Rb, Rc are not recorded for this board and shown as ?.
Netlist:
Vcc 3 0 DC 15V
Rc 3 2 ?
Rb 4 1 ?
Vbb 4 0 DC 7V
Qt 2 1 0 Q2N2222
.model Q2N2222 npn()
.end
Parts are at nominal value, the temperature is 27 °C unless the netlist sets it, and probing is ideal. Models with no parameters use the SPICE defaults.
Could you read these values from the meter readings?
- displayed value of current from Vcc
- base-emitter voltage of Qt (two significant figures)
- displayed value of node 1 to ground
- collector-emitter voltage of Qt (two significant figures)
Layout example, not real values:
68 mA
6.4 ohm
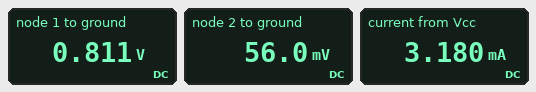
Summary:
3.180 mA
810 mV
0.811 V
56 mV
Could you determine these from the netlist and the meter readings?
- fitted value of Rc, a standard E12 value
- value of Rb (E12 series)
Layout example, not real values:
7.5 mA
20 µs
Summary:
4.7 kΩ
12 kΩ
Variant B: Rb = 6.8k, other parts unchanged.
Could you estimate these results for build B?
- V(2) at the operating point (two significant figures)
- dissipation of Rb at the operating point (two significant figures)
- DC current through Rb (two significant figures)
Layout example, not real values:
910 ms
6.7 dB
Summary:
45 mV
5.6 mW
910 µA
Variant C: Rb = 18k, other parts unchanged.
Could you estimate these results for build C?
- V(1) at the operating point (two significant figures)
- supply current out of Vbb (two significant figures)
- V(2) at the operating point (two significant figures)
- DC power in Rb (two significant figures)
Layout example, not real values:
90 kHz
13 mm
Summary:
810 mV
340 µA
65 mV
2.1 mW
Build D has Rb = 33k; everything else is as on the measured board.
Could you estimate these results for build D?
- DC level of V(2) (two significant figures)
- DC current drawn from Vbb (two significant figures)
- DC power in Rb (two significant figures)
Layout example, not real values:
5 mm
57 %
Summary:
81 mV
190 µA
1.2 mW
